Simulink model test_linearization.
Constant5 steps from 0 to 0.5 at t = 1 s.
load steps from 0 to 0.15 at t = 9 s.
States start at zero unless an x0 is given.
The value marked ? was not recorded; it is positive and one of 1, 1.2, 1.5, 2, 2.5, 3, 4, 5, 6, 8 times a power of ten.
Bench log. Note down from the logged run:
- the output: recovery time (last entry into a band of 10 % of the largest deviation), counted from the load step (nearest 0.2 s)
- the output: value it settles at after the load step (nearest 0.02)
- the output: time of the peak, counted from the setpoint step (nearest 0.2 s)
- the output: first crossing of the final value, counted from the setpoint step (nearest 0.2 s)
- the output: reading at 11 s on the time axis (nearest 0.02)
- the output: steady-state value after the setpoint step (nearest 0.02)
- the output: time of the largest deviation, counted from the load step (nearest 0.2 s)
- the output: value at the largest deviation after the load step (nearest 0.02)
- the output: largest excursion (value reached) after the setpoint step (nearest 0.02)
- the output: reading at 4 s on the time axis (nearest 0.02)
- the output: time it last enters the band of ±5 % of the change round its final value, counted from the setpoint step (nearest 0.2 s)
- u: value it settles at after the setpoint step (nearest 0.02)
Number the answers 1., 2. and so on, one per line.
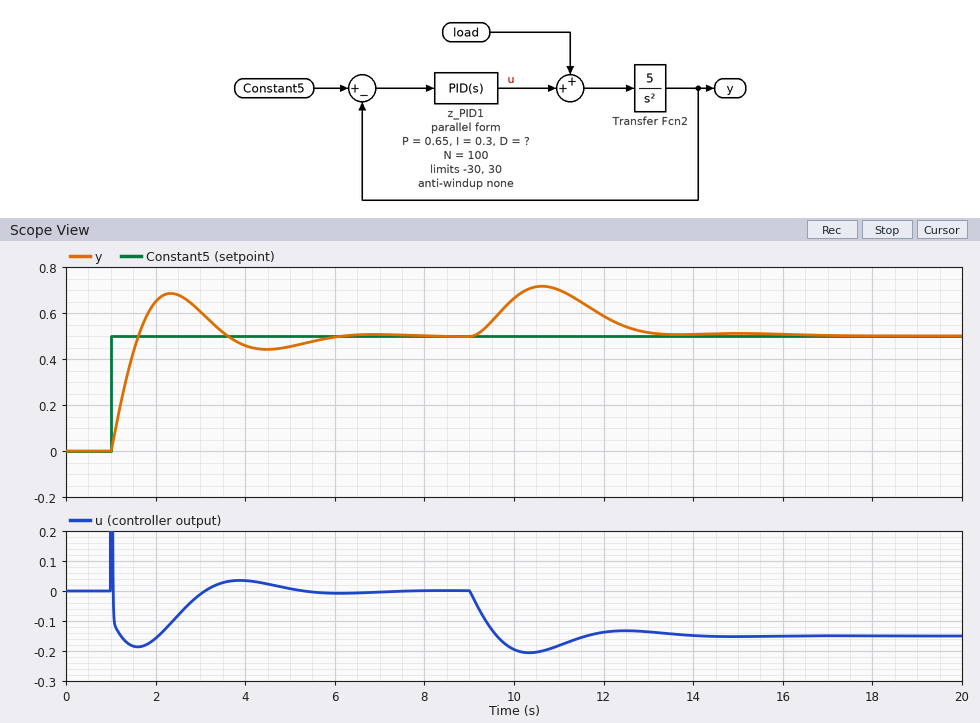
1. 3.8 s
2. 0.50
3. 1.4 s
4. 0.6 s
5. 0.70
6. 0.50
7. 1.6 s
8. 0.72
9. 0.68
10. 0.46
11. 4.4 s
12. 0.00
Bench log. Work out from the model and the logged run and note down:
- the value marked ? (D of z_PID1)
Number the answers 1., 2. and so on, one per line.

1. 0.4
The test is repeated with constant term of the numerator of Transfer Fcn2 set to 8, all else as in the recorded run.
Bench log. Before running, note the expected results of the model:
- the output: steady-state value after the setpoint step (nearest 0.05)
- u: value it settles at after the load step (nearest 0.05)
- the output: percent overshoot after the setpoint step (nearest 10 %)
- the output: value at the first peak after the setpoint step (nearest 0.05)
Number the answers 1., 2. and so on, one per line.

1. 0.50
2. -0.15
3. 30 %
4. 0.65
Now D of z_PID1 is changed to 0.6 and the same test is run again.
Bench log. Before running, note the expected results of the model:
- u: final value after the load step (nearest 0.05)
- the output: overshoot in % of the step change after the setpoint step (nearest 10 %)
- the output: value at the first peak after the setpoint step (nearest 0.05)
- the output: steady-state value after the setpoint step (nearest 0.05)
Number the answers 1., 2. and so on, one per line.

1. -0.15
2. 20 %
3. 0.60
4. 0.50
